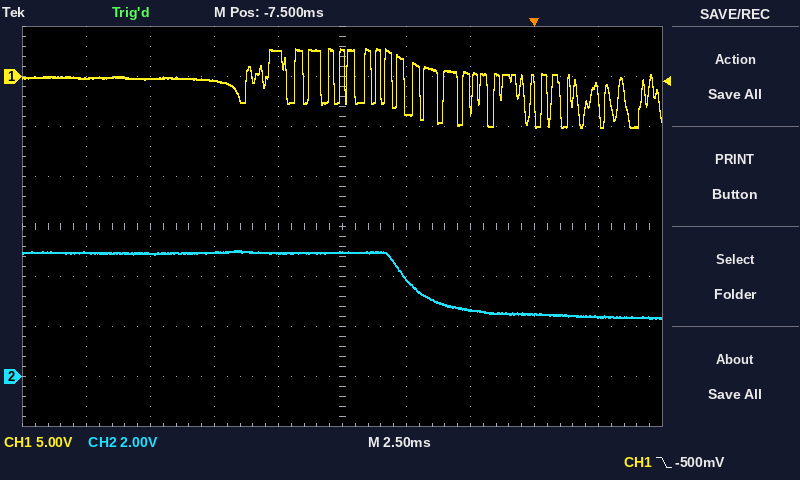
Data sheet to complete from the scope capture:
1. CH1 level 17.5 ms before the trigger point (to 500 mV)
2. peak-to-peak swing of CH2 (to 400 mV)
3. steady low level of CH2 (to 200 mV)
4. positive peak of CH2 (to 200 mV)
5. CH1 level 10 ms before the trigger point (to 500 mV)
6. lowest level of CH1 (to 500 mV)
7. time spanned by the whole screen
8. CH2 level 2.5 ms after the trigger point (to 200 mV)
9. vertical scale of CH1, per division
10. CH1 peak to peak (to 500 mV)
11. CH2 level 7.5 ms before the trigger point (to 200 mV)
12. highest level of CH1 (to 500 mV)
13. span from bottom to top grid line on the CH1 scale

0.0 V
2.8 V
2.4 V
5.0 V
2.5 V
-5.0 V
25 ms
2.4 V
5 V
8.0 V
5.0 V
3.0 V
40 V
